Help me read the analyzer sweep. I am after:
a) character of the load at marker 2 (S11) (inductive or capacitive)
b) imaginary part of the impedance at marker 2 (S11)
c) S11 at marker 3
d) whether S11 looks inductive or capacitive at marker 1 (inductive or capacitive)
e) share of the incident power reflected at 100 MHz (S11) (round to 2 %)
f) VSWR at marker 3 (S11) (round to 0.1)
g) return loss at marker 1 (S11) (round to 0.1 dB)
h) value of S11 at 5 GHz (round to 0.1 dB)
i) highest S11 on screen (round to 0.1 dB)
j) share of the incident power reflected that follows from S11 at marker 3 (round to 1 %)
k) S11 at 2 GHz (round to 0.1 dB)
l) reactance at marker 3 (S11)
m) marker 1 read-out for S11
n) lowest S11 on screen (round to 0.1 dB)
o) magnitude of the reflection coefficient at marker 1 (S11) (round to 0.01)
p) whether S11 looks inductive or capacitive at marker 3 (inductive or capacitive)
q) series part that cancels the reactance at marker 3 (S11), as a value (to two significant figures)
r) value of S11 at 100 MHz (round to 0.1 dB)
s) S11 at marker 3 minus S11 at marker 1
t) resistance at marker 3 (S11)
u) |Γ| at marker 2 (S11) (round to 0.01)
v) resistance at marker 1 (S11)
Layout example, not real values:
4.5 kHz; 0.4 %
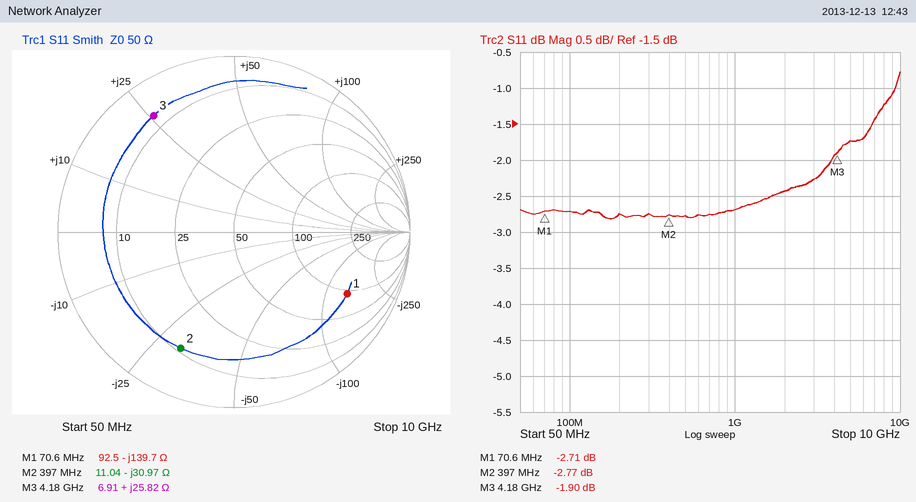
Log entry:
capacitive; -30.97 Ω; -1.90 dB; capacitive; 54 %; 9.2; 2.7 dB; -1.7 dB; -0.8 dB; 65 %; -2.4 dB; +25.82 Ω; -2.71 dB; -2.8 dB; 0.73; inductive; 1.5 pF; -2.7 dB; 0.81 dB; 6.91 Ω; 0.73; 92.5 Ω
